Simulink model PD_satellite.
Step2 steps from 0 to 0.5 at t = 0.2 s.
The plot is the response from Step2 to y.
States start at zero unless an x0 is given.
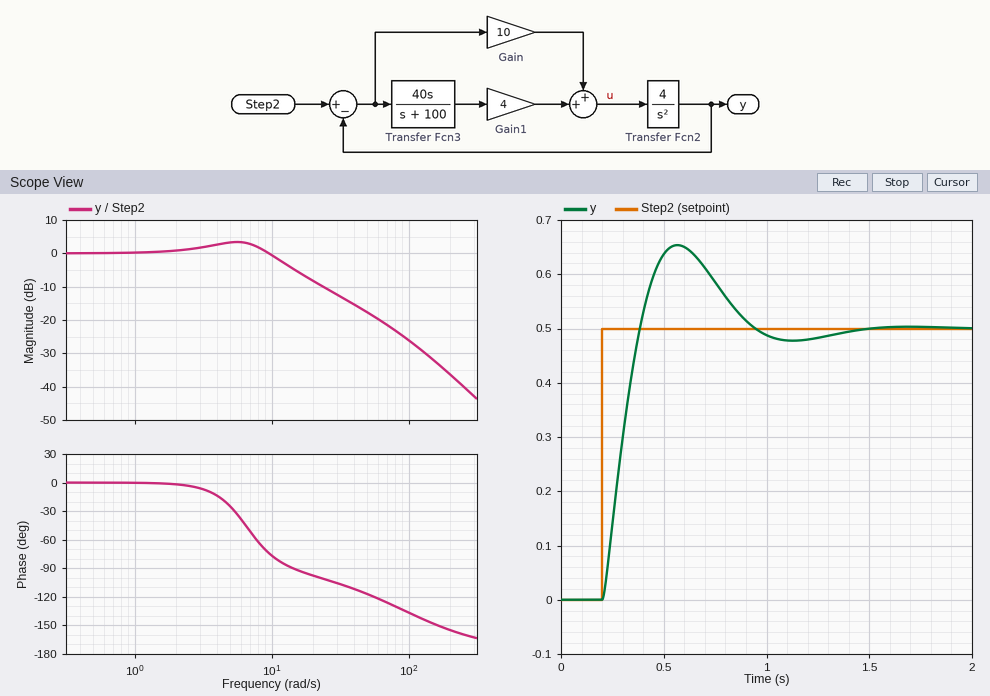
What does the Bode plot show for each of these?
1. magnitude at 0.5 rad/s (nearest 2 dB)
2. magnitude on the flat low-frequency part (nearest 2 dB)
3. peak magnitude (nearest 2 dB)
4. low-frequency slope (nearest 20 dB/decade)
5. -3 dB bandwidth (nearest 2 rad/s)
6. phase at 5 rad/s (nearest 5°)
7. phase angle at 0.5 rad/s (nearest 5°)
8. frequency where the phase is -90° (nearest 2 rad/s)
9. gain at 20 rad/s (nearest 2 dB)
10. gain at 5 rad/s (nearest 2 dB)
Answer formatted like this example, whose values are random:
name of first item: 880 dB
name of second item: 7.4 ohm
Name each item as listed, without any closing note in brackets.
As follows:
magnitude at 0.5 rad/s: 0 dB
magnitude on the flat low-frequency part: 0 dB
peak magnitude: 4 dB
low-frequency slope: 0 dB/decade
-3 dB bandwidth: 12 rad/s
phase at 5 rad/s: -25°
phase angle at 0.5 rad/s: 0°
frequency where the phase is -90°: 14 rad/s
gain at 20 rad/s: -8 dB
gain at 5 rad/s: 4 dB
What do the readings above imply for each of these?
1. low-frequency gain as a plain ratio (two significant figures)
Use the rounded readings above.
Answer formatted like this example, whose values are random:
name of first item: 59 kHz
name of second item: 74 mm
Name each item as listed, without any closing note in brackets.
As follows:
low-frequency gain as a plain ratio: 1.0
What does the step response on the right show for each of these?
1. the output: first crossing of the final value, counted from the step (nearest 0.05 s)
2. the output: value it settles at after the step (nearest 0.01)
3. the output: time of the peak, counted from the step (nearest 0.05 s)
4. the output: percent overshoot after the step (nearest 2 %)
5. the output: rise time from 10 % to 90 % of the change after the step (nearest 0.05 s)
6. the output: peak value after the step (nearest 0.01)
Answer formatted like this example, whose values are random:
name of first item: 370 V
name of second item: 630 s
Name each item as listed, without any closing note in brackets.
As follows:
the output: first crossing of the final value, counted from the step: 0.20 s
the output: value it settles at after the step: 0.50
the output: time of the peak, counted from the step: 0.35 s
the output: percent overshoot after the step: 30 %
the output: rise time from 10 % to 90 % of the change after the step: 0.15 s
the output: peak value after the step: 0.65
